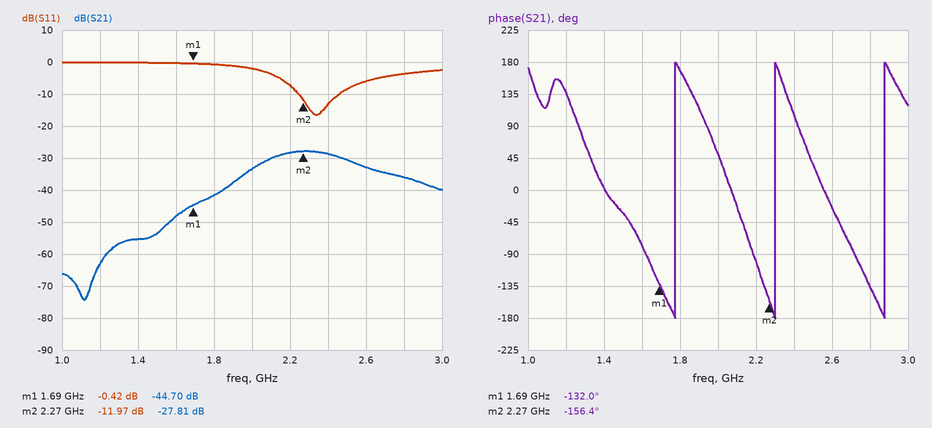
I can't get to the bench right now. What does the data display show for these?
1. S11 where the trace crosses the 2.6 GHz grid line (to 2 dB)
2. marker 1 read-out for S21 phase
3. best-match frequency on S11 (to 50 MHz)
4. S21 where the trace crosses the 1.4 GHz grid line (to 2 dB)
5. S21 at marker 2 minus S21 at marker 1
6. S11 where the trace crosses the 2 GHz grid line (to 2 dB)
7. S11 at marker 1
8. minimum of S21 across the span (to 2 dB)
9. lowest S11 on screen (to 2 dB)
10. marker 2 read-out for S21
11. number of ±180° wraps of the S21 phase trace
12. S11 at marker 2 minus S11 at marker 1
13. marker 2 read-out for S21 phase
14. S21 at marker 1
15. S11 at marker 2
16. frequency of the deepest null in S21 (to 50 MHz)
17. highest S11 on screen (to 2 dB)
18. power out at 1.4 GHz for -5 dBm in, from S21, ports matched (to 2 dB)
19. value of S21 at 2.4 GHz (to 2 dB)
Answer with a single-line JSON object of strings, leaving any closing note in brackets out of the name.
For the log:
{"S11 where the trace crosses the 2.6 GHz grid line": "-6 dB", "marker 1 read-out for S21 phase": "-132.0°", "best-match frequency on S11": "2.35 GHz", "S21 where the trace crosses the 1.4 GHz grid line": "-56 dB", "S21 at marker 2 minus S21 at marker 1": "16.89 dB", "S11 where the trace crosses the 2 GHz grid line": "-2 dB", "S11 at marker 1": "-0.42 dB", "minimum of S21 across the span": "-74 dB", "lowest S11 on screen": "-16 dB", "marker 2 read-out for S21": "-27.81 dB", "number of ±180° wraps of the S21 phase trace": "3", "S11 at marker 2 minus S11 at marker 1": "-11.55 dB", "marker 2 read-out for S21 phase": "-156.4°", "S21 at marker 1": "-44.70 dB", "S11 at marker 2": "-11.97 dB", "frequency of the deepest null in S21": "1.10 GHz", "highest S11 on screen": "0 dB", "power out at 1.4 GHz for -5 dBm in, from S21, ports matched": "-60 dBm", "value of S21 at 2.4 GHz": "-28 dB"}
